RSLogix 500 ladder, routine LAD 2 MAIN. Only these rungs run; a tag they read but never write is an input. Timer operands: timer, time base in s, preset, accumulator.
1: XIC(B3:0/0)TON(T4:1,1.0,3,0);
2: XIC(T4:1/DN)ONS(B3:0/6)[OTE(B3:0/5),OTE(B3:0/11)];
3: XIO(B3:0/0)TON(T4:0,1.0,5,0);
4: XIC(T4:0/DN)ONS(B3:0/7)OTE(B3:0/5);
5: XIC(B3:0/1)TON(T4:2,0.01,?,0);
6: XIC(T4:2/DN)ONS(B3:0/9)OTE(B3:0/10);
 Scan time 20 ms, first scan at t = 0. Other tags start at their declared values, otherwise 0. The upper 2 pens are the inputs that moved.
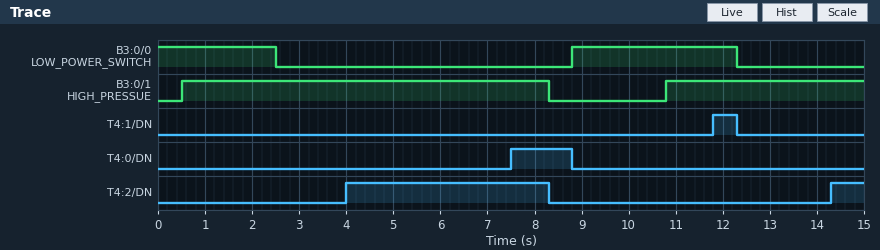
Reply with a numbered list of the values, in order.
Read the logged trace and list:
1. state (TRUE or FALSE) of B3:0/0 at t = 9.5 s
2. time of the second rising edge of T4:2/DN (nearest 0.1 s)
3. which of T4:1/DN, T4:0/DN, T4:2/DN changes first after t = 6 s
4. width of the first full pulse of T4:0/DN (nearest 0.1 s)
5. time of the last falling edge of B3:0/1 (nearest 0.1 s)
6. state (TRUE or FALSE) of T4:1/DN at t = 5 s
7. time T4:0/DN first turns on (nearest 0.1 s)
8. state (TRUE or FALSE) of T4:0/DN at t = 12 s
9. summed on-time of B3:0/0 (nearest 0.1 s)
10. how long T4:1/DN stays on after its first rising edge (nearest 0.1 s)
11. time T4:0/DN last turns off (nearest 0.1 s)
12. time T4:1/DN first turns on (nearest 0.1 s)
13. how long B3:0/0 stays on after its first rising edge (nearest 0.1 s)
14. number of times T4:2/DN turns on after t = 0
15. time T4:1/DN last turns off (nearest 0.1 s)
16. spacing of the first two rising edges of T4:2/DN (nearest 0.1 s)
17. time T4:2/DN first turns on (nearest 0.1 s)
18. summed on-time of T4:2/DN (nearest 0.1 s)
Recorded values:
1. TRUE
2. 14.3 s
3. T4:0/DN
4. 1.3 s
5. 8.3 s
6. FALSE
7. 7.5 s
8. FALSE
9. 6.0 s
10. 0.5 s
11. 8.8 s
12. 11.8 s
13. 3.5 s
14. 2
15. 12.3 s
16. 10.3 s
17. 4.0 s
18. 5.0 s
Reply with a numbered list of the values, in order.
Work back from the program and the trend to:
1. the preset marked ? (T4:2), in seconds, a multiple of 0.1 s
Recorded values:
1. 3.5 s
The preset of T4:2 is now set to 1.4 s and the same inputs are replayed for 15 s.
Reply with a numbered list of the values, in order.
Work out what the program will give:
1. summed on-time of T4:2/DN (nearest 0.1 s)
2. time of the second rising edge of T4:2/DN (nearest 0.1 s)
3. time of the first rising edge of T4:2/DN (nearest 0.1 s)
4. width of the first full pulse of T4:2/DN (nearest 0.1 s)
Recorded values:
1. 9.2 s
2. 12.2 s
3. 1.9 s
4. 6.4 s
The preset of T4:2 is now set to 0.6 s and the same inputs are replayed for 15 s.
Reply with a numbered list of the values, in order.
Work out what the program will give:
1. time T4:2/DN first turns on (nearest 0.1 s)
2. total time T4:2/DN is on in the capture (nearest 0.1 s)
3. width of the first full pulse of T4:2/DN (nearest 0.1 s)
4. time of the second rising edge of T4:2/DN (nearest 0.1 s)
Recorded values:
1. 1.1 s
2. 10.8 s
3. 7.2 s
4. 11.4 s
